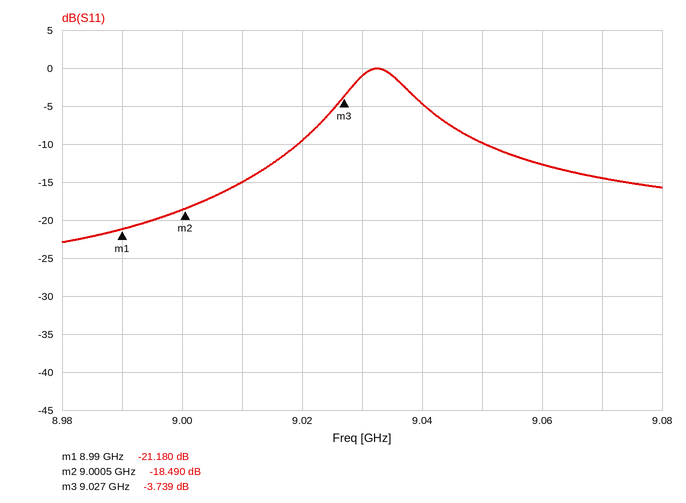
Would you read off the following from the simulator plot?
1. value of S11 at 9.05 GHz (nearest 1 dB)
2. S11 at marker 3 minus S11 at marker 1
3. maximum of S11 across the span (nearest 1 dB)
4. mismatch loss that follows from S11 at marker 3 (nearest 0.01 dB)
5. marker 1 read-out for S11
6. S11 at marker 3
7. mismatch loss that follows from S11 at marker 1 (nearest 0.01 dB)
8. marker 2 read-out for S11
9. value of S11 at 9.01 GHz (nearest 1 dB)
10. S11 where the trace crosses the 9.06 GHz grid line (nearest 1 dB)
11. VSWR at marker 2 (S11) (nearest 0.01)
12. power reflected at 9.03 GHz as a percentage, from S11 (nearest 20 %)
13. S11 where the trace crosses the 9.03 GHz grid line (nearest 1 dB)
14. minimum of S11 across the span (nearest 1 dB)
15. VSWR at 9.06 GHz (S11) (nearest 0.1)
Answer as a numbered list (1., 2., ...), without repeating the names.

1. -10 dB
2. 17.441 dB
3. 0 dB
4. 2.39 dB
5. -21.180 dB
6. -3.739 dB
7. 0.03 dB
8. -18.490 dB
9. -15 dB
10. -13 dB
11. 1.27
12. 80 %
13. -1 dB
14. -23 dB
15. 1.6
